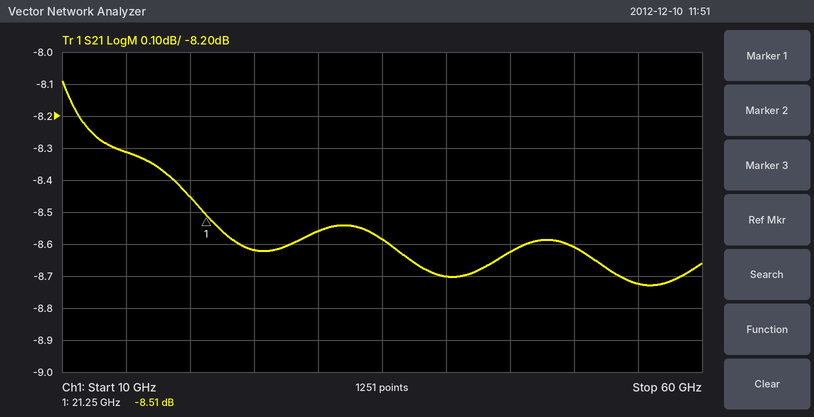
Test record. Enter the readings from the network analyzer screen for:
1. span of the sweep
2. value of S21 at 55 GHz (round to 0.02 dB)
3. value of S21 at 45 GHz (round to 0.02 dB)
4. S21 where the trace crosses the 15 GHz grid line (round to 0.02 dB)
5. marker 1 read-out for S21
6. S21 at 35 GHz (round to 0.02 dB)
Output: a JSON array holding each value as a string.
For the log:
["50 GHz", "-8.72 dB", "-8.62 dB", "-8.32 dB", "-8.51 dB", "-8.58 dB"]
